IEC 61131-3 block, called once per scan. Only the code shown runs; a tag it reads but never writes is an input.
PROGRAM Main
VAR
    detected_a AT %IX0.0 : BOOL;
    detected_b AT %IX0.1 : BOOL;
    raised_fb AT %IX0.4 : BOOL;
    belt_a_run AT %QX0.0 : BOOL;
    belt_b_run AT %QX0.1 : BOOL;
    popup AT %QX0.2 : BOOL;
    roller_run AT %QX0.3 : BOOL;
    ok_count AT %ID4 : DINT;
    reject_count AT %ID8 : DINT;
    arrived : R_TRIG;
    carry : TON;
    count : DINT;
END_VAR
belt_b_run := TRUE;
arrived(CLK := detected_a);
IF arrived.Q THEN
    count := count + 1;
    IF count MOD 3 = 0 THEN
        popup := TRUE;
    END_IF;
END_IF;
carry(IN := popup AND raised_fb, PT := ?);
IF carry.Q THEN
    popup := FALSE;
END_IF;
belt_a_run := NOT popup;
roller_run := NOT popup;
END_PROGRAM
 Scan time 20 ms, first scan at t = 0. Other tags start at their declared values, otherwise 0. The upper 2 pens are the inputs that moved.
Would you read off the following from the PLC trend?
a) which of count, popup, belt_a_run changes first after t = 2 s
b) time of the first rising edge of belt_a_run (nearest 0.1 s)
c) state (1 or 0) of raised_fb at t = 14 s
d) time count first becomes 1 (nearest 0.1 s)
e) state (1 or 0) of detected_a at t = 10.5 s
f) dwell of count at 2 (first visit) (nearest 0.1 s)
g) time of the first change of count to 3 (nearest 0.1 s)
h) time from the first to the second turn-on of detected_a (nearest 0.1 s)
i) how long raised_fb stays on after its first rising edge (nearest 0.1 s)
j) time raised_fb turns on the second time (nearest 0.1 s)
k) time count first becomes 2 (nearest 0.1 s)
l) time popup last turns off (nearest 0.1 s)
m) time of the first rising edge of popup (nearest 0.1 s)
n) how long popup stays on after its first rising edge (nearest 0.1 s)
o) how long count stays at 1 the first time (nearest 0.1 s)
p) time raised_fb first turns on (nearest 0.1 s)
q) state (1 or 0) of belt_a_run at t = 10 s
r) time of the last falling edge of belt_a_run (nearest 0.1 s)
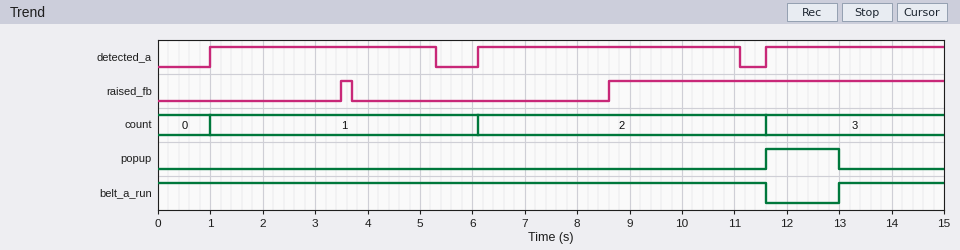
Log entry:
count
13.0 s
1
1.0 s
1
5.5 s
11.6 s
5.1 s
0.2 s
8.6 s
6.1 s
13.0 s
11.6 s
1.4 s
5.1 s
3.5 s
1
11.6 s
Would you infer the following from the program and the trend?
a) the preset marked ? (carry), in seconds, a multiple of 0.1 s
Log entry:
1.4 s
